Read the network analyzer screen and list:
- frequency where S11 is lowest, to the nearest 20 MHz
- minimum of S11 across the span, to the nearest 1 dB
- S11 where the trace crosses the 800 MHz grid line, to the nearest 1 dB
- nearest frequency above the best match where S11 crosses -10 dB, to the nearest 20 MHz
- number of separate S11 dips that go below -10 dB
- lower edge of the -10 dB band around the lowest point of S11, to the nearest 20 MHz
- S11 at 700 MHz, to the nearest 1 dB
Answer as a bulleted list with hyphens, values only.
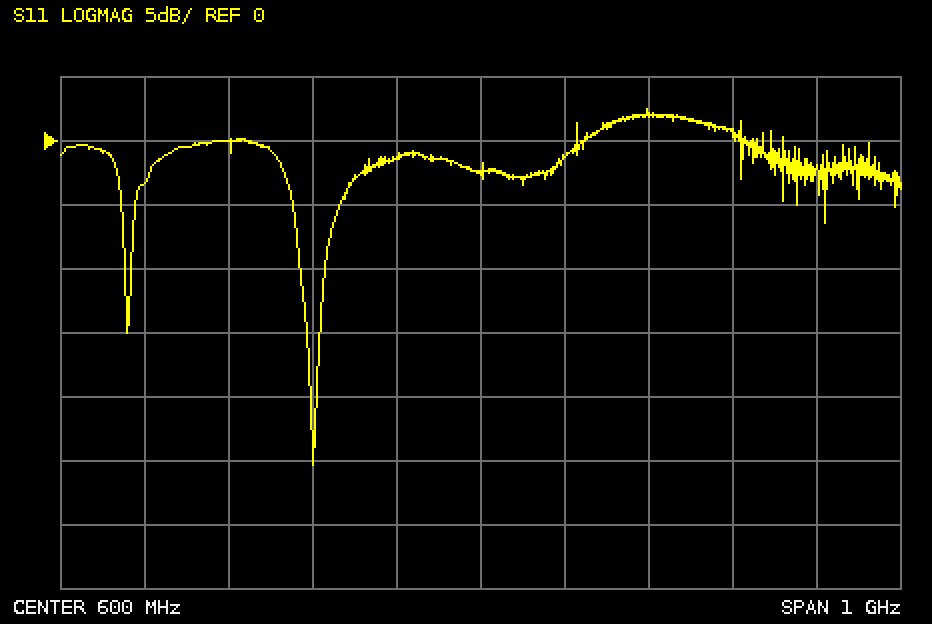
- 400 MHz
- -25 dB
- 2 dB
- 420 MHz
- 2
- 380 MHz
- -1 dB
